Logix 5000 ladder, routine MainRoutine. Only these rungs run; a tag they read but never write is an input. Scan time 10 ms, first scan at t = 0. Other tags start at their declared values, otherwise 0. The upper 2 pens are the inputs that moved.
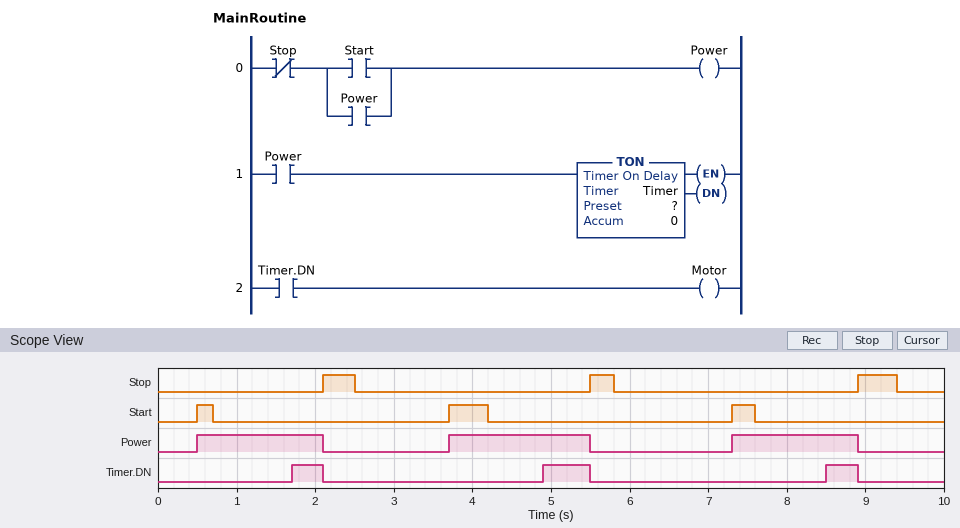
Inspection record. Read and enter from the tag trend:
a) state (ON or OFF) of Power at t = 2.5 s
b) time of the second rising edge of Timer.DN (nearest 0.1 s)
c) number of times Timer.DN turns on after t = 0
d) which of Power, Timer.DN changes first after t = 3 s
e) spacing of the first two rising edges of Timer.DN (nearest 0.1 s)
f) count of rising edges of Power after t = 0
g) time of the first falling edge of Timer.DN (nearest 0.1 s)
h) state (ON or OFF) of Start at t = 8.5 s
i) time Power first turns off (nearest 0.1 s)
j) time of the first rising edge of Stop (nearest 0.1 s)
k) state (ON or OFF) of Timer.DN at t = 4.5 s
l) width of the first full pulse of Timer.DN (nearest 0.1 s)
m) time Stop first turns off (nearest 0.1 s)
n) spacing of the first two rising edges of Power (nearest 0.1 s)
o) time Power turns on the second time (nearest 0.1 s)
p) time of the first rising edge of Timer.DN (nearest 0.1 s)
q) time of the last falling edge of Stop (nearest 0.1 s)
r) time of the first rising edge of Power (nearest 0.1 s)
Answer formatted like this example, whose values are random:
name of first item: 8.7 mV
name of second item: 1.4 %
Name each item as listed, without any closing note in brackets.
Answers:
state (ON or OFF) of Power at t = 2.5 s: OFF
time of the second rising edge of Timer.DN: 4.9 s
number of times Timer.DN turns on after t = 0: 3
which of Power, Timer.DN changes first after t = 3 s: Power
spacing of the first two rising edges of Timer.DN: 3.2 s
count of rising edges of Power after t = 0: 3
time of the first falling edge of Timer.DN: 2.1 s
state (ON or OFF) of Start at t = 8.5 s: OFF
time Power first turns off: 2.1 s
time of the first rising edge of Stop: 2.1 s
state (ON or OFF) of Timer.DN at t = 4.5 s: OFF
width of the first full pulse of Timer.DN: 0.4 s
time Stop first turns off: 2.5 s
spacing of the first two rising edges of Power: 3.2 s
time Power turns on the second time: 3.7 s
time of the first rising edge of Timer.DN: 1.7 s
time of the last falling edge of Stop: 9.4 s
time of the first rising edge of Power: 0.5 s
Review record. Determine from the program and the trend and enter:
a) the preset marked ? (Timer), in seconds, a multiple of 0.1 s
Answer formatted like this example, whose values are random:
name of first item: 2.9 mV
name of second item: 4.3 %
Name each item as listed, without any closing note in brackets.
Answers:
the preset marked ? (Timer), in seconds, a multiple of 0.1 s: 1.2 s
